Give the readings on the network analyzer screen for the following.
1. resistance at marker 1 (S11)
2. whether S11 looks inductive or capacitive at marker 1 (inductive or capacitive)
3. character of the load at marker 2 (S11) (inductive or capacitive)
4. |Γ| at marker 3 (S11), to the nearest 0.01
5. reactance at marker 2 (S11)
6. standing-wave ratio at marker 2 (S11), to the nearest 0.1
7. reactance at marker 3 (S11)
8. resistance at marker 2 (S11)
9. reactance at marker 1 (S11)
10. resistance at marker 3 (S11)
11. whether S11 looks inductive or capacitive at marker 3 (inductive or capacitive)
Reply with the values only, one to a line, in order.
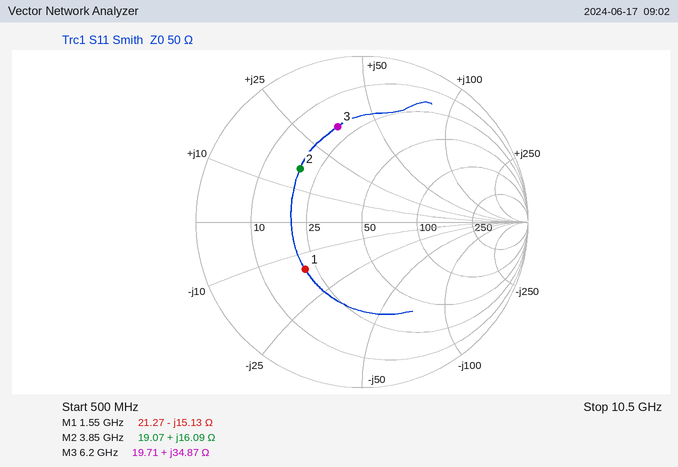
21.27 Ω
capacitive
inductive
0.59
+16.09 Ω
2.9
+34.87 Ω
19.07 Ω
-15.13 Ω
19.71 Ω
inductive
